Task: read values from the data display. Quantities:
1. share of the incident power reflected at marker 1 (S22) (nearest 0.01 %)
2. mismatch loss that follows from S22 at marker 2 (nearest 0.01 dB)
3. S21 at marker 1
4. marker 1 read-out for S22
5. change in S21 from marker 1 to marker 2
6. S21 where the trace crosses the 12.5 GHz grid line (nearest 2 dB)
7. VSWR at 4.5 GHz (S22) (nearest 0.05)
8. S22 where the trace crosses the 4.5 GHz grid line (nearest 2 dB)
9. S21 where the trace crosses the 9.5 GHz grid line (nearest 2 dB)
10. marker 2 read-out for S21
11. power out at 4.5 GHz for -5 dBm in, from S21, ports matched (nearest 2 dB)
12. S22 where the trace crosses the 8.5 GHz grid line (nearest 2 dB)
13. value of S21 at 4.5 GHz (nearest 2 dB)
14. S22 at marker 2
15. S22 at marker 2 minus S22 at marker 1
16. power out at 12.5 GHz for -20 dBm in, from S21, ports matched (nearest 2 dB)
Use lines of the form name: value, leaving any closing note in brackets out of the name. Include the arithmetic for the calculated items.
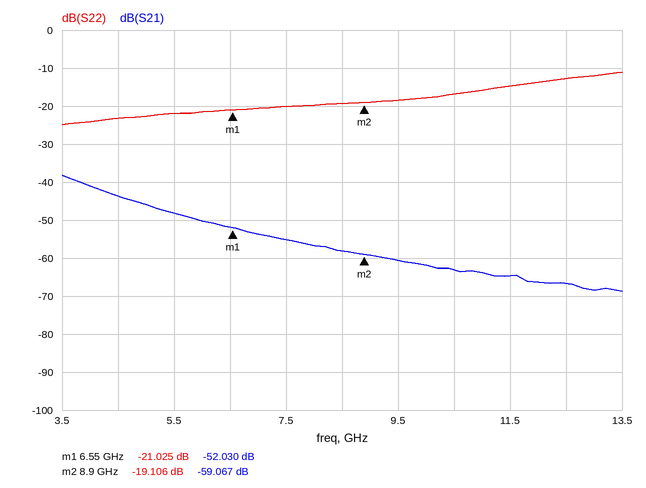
share of the incident power reflected at marker 1 (S22): 10^(-21.025/10) ≈ 0.79 %
mismatch loss that follows from S22 at marker 2: −10 log10(1 − 10^(-19.106/10)) ≈ 0.05 dB
S21 at marker 1: -52.030 dB
marker 1 read-out for S22: -21.025 dB
change in S21 from marker 1 to marker 2: -59.067 − (-52.03) = -7.037 dB
S21 where the trace crosses the 12.5 GHz grid line: -66 dB
VSWR at 4.5 GHz (S22): |Γ| = 10^(-24/20) = 0.0631; VSWR = (1 + 0.0631)/(1 − 0.0631) ≈ 1.13, so 1.15 to the nearest 0.05
S22 where the trace crosses the 4.5 GHz grid line: -24 dB
S21 where the trace crosses the 9.5 GHz grid line: -60 dB
marker 2 read-out for S21: -59.067 dB
power out at 4.5 GHz for -5 dBm in, from S21, ports matched: -5 dBm + (-44 dB) = -48 dBm
S22 where the trace crosses the 8.5 GHz grid line: -20 dB
value of S21 at 4.5 GHz: -44 dB
S22 at marker 2: -19.106 dB
S22 at marker 2 minus S22 at marker 1: -19.106 − (-21.025) = 1.919 dB
power out at 12.5 GHz for -20 dBm in, from S21, ports matched: -20 dBm + (-66 dB) = -86 dBm
